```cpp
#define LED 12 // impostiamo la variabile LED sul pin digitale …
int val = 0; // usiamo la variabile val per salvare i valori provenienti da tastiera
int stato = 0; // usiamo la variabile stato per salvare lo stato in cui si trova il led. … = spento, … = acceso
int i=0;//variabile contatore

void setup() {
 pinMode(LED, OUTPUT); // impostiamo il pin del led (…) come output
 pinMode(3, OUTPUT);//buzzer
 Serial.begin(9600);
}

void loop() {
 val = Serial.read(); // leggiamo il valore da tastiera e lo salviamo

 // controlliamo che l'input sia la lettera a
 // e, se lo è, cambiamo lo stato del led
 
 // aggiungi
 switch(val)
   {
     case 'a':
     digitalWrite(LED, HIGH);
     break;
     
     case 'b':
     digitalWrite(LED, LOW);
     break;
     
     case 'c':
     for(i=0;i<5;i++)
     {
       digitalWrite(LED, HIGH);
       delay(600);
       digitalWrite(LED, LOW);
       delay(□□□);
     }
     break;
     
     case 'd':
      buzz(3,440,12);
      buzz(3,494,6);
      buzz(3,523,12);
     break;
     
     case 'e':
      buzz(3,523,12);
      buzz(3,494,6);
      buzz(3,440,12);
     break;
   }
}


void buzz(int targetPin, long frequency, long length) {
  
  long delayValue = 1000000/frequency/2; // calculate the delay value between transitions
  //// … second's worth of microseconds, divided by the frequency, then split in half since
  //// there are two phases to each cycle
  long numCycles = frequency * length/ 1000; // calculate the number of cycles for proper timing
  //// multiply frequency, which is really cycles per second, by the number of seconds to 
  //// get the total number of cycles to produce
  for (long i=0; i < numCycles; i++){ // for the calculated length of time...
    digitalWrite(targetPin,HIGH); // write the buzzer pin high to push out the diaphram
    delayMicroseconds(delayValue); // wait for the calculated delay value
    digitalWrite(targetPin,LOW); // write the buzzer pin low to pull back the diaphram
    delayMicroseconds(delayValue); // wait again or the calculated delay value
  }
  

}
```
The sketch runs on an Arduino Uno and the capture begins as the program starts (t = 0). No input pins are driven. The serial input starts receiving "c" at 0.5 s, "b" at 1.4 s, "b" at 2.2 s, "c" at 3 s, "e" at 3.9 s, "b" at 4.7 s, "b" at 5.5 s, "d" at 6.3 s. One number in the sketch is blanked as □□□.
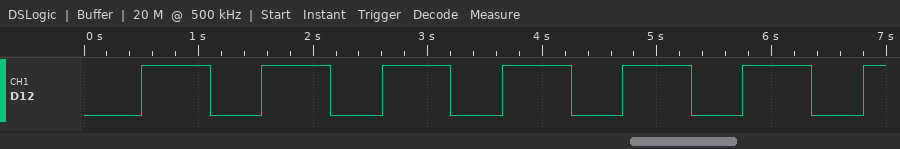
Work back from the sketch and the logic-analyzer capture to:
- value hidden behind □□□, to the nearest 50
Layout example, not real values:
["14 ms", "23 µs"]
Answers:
["450"]
